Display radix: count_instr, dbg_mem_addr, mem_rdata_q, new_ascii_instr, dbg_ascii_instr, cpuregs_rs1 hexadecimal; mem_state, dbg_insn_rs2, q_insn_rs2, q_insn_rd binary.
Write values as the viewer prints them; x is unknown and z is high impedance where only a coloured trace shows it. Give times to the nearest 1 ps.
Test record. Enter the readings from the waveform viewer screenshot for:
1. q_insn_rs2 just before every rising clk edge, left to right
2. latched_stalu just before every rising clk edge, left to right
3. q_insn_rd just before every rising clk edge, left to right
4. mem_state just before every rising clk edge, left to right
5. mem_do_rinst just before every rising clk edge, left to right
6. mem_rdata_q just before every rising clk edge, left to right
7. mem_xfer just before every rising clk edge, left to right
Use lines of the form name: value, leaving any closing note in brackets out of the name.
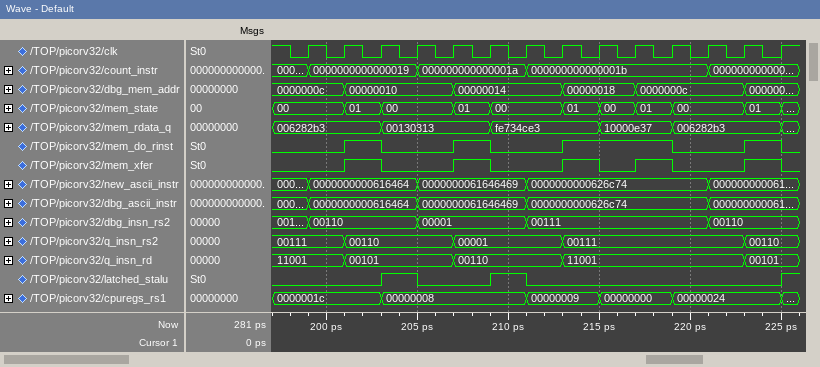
q_insn_rs2 just before every rising clk edge, left to right: 00111, 00111, 00110, 00110, 00110, 00001, 00001, 00001, 00111, 00111, 00111, 00111, 00111, 00110
latched_stalu just before every rising clk edge, left to right: 0 0 0 1 0 0 1 0 0 0 0 0 0 0
q_insn_rd just before every rising clk edge, left to right: 11001, 11001, 00101, 00101, 00101, 00110, 00110, 00110, 11001, 11001, 11001, 11001, 11001, 00101
mem_state just before every rising clk edge, left to right: 00, 00, 01, 00, 00, 01, 00, 00, 01, 00, 01, 00, 00, 01
mem_do_rinst just before every rising clk edge, left to right: 0 0 1 0 0 1 0 0 1 1 1 0 0 1
mem_rdata_q just before every rising clk edge, left to right: 006282b3, 006282b3, 006282b3, 00130313, 00130313, 00130313, fe734ce3, fe734ce3, fe734ce3, 10000e37, 10000e37, 006282b3, 006282b3, 006282b3
mem_xfer just before every rising clk edge, left to right: 0 0 1 0 0 1 0 0 1 0 1 0 0 1
